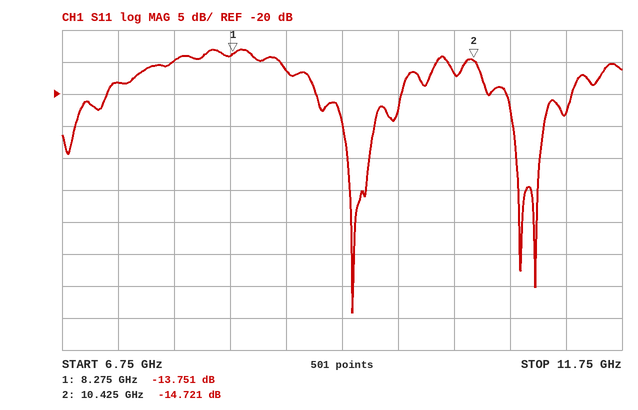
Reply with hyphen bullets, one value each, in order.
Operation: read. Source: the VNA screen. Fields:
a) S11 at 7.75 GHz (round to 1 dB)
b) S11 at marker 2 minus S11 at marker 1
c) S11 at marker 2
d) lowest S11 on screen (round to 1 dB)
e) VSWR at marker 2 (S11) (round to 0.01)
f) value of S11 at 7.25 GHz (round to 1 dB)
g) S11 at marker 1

- -15 dB
- -0.970 dB
- -14.721 dB
- -54 dB
- 1.45
- -18 dB
- -13.751 dB
